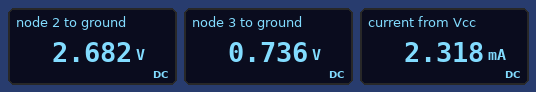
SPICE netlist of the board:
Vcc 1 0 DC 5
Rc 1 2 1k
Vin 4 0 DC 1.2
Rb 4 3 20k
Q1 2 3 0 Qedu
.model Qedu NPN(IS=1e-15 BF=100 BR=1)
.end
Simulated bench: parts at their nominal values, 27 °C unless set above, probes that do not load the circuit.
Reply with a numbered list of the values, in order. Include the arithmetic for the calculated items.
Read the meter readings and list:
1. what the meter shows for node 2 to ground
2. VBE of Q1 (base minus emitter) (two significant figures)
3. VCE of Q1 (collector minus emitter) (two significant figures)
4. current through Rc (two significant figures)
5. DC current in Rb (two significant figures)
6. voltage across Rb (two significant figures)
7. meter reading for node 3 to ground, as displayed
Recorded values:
1. 2.682 V
2. 736 mV = 740 mV
3. 2.682 V = 2.7 V
4. (5 V - 2.682 V) / 1 kΩ = 2.3 mA
5. (1.2 V - 736 mV) / 20 kΩ = 23 µA
6. 1.2 V - 736 mV = 460 mV
7. 0.736 V
